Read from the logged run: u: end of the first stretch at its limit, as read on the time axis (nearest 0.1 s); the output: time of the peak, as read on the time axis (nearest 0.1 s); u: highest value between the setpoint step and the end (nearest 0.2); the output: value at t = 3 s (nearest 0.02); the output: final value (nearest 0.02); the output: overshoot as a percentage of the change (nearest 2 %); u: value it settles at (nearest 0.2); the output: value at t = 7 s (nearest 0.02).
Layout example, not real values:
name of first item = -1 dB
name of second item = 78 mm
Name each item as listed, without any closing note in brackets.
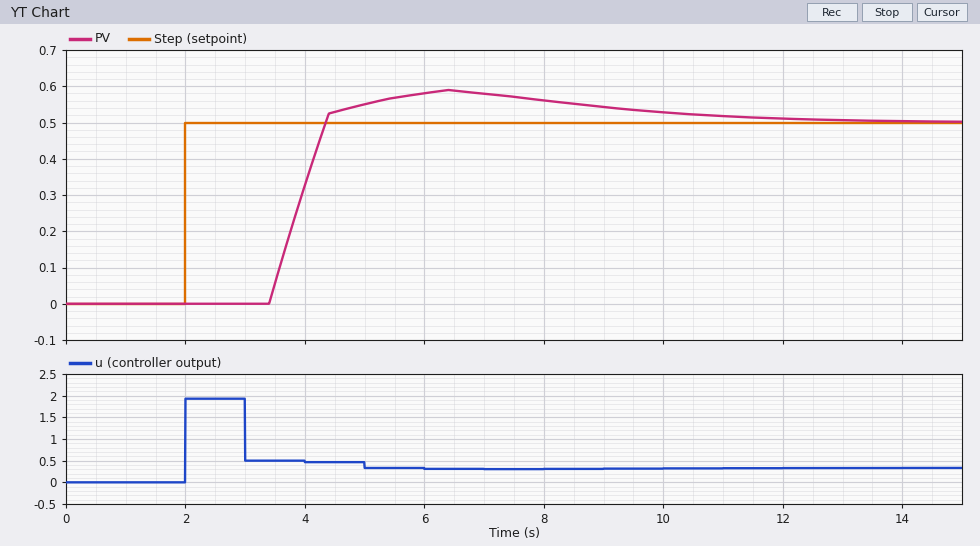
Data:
u: end of the first stretch at its limit, as read on the time axis = 3.0 s
the output: time of the peak, as read on the time axis = 6.4 s
u: highest value between the setpoint step and the end = 2.0
the output: value at t = 3 s = 0.00
the output: final value = 0.50
the output: overshoot as a percentage of the change = 18 %
u: value it settles at = 0.4
the output: value at t = 7 s = 0.58
